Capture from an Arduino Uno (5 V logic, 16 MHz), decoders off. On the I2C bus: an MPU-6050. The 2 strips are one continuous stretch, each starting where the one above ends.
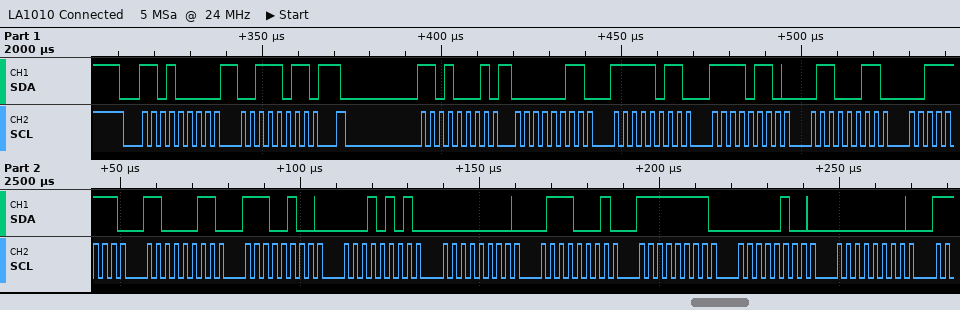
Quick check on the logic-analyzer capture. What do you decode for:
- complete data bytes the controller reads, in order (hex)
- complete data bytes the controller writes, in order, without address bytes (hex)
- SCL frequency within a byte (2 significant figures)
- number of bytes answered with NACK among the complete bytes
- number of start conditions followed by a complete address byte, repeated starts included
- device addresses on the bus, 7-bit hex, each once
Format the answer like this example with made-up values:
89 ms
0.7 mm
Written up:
03 FB F6 63 3F C3 E4 15 00 71 FF 04 00
3B
400 kHz
0
2
0x68
